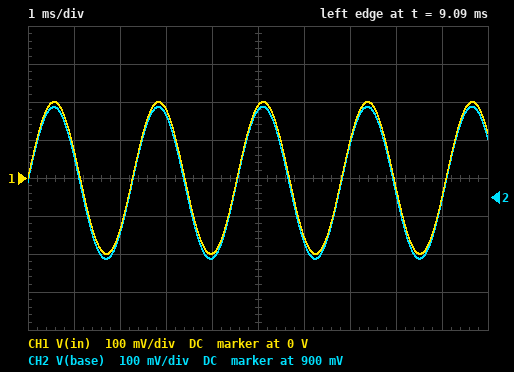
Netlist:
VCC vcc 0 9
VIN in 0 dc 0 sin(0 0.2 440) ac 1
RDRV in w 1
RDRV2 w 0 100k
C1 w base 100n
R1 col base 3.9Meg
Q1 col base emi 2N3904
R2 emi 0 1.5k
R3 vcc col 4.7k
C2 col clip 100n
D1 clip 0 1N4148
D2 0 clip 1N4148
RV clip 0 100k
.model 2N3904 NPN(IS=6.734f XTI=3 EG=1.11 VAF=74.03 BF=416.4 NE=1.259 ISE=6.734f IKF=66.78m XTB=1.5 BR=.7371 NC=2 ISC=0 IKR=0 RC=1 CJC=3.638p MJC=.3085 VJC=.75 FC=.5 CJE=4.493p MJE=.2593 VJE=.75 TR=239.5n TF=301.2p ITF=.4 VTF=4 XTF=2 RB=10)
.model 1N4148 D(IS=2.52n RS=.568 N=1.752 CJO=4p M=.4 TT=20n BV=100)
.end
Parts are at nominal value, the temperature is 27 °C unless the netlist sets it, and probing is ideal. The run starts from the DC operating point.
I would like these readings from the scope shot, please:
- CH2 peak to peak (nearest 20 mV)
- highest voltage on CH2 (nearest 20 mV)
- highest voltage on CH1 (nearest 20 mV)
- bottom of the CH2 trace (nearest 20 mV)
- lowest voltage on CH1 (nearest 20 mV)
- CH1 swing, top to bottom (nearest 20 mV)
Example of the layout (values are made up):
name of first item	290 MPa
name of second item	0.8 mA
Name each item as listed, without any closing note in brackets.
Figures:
CH2 peak to peak	400 mV
highest voltage on CH2	1.14 V
highest voltage on CH1	200 mV
bottom of the CH2 trace	740 mV
lowest voltage on CH1	-200 mV
CH1 swing, top to bottom	400 mV
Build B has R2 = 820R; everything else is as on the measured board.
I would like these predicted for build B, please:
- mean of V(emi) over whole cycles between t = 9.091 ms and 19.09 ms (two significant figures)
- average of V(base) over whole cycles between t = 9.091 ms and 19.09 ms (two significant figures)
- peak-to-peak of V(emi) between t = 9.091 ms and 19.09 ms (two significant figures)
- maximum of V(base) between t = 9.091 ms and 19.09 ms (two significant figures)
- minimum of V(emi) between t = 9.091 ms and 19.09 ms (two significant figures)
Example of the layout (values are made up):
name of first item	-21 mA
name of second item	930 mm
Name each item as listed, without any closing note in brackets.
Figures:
mean of V(emi) over whole cycles between t = 9.091 ms and 19.09 ms	180 mV
average of V(base) over whole cycles between t = 9.091 ms and 19.09 ms	800 mV
peak-to-peak of V(emi) between t = 9.091 ms and 19.09 ms	330 mV
maximum of V(base) between t = 9.091 ms and 19.09 ms	1.0 V
minimum of V(emi) between t = 9.091 ms and 19.09 ms	24 mV
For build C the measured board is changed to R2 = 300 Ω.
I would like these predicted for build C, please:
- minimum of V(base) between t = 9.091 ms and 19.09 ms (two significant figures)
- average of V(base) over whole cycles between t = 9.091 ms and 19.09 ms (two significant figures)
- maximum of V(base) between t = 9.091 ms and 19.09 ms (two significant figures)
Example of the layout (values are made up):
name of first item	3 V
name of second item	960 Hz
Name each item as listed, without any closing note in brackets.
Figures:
minimum of V(base) between t = 9.091 ms and 19.09 ms	450 mV
average of V(base) over whole cycles between t = 9.091 ms and 19.09 ms	650 mV
maximum of V(base) between t = 9.091 ms and 19.09 ms	860 mV
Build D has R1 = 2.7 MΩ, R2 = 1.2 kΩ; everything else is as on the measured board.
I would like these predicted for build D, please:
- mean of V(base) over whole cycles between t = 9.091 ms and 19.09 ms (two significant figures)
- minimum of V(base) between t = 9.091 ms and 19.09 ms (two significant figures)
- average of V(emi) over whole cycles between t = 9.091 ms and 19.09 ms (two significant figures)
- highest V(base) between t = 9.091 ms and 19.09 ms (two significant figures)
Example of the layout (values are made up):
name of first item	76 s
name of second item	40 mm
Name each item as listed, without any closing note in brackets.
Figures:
mean of V(base) over whole cycles between t = 9.091 ms and 19.09 ms	990 mV
minimum of V(base) between t = 9.091 ms and 19.09 ms	790 mV
average of V(emi) over whole cycles between t = 9.091 ms and 19.09 ms	360 mV
highest V(base) between t = 9.091 ms and 19.09 ms	1.2 V
